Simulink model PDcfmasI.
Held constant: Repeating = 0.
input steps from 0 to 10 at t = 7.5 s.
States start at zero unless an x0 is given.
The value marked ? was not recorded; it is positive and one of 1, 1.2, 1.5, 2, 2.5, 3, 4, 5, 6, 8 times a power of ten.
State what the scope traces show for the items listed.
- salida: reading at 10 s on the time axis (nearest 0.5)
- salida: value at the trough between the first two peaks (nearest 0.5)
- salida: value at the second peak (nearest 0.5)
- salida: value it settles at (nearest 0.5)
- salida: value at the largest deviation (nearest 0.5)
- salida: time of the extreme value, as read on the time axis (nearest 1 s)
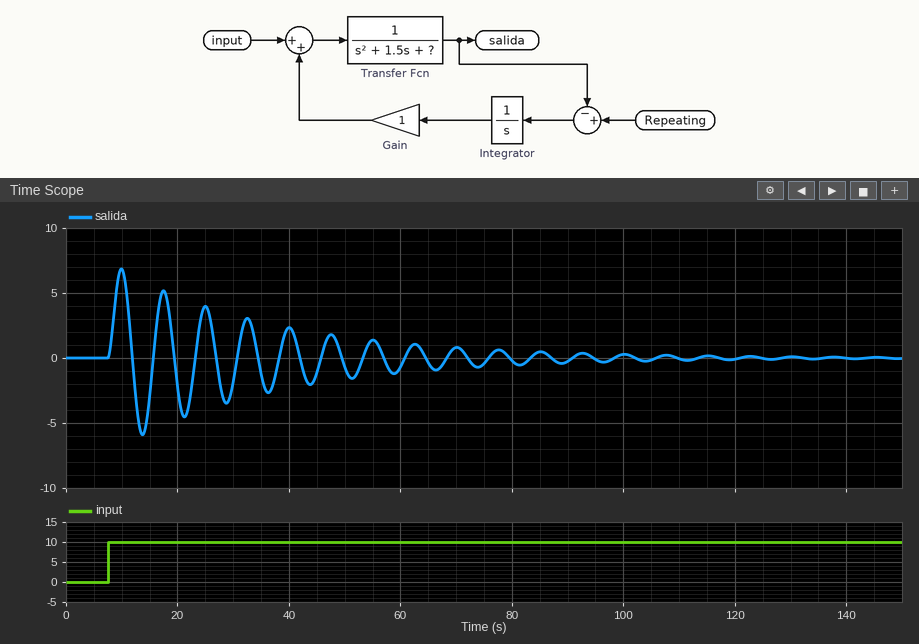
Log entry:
7.0
-6.0
5.0
0.0
7.0
10 s
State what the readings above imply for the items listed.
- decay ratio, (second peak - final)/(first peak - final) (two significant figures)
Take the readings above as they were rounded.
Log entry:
0.71
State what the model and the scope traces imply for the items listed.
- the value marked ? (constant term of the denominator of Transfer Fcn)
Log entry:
0.8
